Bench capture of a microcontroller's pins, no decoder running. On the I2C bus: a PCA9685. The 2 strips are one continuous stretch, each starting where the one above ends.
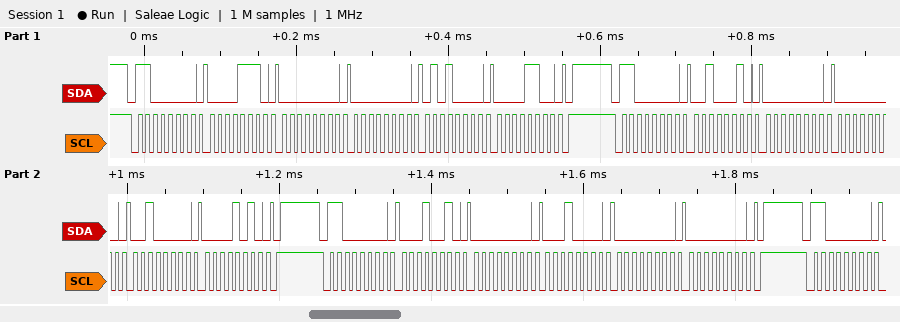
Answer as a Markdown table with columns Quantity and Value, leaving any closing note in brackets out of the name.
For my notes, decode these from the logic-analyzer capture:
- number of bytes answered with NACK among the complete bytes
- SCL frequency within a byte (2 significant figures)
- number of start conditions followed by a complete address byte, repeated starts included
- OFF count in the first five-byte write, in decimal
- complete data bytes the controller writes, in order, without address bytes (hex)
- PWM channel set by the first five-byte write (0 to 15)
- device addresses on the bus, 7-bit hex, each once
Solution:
| Quantity | Value |
|---|---|
| number of bytes answered with NACK among the complete bytes | 0 |
| SCL frequency within a byte | 100 kHz |
| number of start conditions followed by a complete address byte, repeated starts included | 4 |
| OFF count in the first five-byte write, in decimal | 3152 |
| complete data bytes the controller writes, in order, without address bytes | 0E 00 00 50 0C 22 00 00 20 0A 12 00 10 00 00 |
| PWM channel set by the first five-byte write | 2 |
| device addresses on the bus, 7-bit hex, each once | 0x60 |
